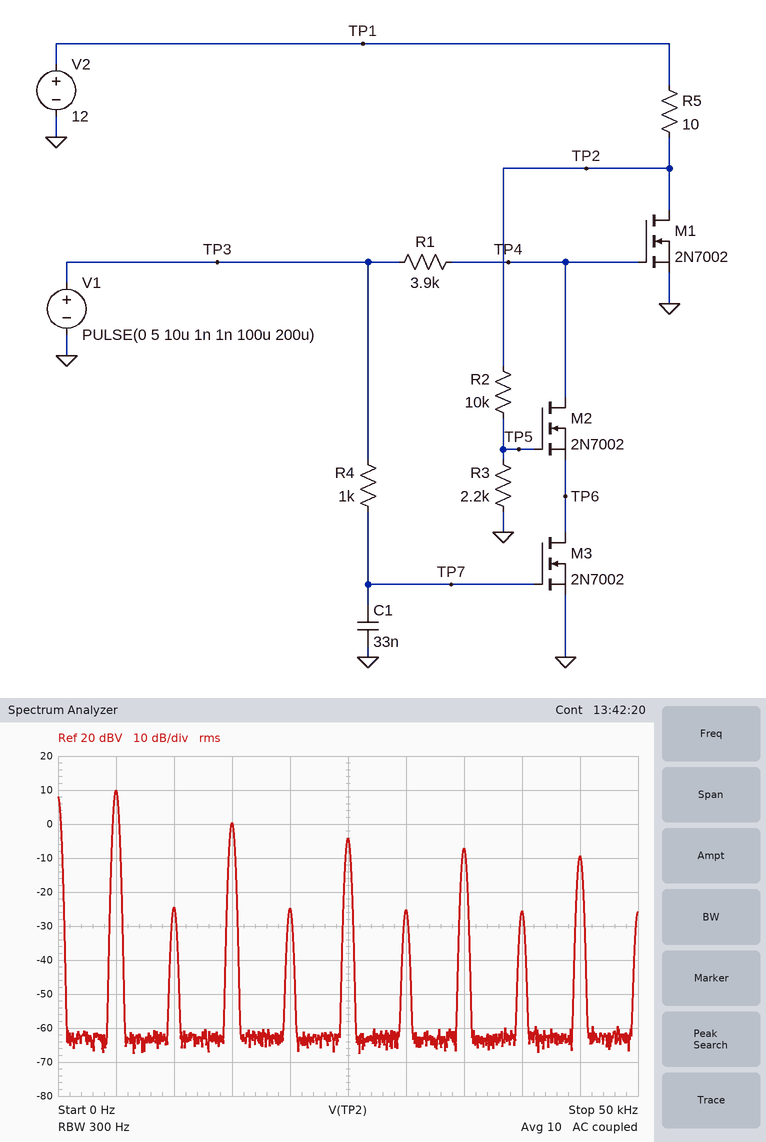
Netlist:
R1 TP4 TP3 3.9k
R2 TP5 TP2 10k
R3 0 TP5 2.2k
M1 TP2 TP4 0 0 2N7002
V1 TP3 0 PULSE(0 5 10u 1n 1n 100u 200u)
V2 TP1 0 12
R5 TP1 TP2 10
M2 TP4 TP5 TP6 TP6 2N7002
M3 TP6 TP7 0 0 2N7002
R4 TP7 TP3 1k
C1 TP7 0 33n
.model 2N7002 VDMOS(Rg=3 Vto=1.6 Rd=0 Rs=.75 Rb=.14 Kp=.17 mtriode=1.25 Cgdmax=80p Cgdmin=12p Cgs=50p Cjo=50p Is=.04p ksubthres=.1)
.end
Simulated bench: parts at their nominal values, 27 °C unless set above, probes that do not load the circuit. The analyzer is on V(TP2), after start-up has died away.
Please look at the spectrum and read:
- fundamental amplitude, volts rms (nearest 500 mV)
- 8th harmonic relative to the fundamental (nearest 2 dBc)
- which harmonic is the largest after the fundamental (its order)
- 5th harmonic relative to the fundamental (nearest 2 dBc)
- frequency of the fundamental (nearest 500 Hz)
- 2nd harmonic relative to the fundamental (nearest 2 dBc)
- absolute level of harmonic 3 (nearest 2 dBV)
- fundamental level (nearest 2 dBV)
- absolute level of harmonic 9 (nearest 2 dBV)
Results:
3.0 V
-36 dBc
3
-14 dBc
5.0 kHz
-34 dBc
0 dBV
10 dBV
-10 dBV
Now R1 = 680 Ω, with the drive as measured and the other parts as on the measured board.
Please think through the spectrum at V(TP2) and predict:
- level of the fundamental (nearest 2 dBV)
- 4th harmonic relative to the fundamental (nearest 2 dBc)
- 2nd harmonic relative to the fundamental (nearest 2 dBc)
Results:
10 dBV
-48 dBc
-48 dBc
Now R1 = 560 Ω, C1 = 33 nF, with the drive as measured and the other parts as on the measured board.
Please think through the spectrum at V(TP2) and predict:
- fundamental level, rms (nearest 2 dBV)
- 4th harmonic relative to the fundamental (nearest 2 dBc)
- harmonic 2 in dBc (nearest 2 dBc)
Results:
10 dBV
-50 dBc
-50 dBc
